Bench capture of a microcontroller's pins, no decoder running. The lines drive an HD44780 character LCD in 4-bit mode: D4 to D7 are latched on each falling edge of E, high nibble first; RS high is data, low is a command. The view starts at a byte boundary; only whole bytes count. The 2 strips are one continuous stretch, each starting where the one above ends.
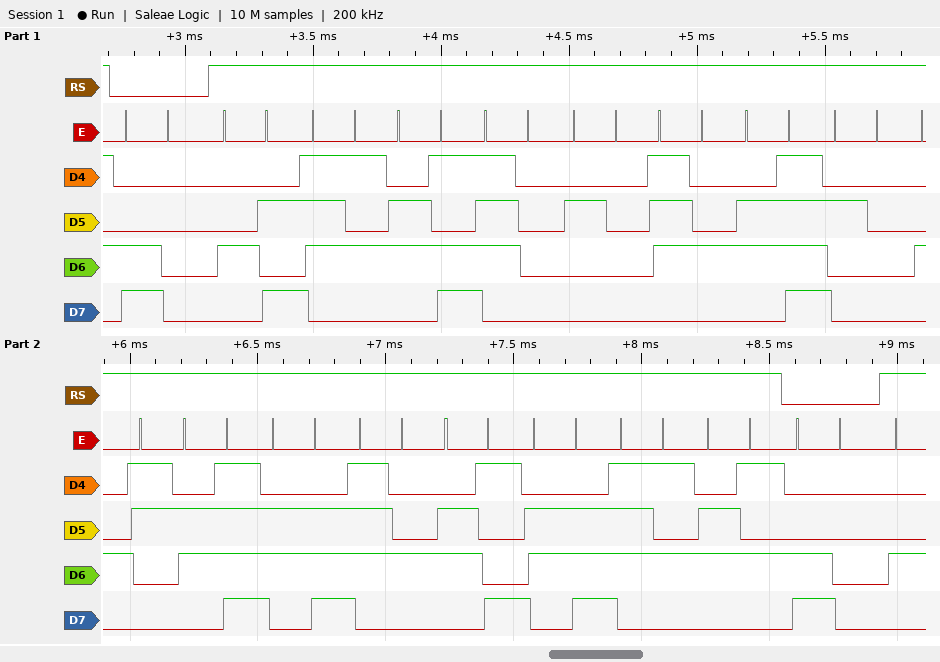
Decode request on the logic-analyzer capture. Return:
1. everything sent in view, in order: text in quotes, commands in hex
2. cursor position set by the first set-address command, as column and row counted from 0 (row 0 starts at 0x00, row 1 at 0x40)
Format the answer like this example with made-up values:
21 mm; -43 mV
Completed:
0xC0 "Jump to Continue" 0xC0; column 0, row 1
